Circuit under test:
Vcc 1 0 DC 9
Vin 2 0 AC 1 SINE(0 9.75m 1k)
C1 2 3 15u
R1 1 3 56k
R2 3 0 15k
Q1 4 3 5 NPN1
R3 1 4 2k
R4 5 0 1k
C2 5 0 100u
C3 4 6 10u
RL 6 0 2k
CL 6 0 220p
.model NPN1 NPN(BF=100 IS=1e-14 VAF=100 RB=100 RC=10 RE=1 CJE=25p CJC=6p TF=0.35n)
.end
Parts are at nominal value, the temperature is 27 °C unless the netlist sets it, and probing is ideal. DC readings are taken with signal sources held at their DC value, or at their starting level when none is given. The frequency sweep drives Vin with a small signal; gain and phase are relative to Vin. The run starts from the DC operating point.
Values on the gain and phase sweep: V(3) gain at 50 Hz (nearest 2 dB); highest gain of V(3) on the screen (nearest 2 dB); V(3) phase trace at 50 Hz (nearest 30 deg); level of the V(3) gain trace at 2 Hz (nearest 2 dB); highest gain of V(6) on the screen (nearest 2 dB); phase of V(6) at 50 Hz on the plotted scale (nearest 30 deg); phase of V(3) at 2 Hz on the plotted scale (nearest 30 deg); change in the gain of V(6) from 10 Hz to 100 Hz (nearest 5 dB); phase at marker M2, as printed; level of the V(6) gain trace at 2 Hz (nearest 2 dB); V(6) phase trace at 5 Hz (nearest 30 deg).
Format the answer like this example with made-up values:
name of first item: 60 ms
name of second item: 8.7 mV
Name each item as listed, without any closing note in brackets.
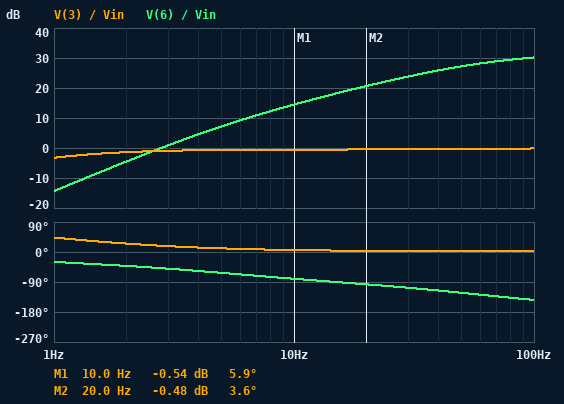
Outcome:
V(3) gain at 50 Hz: 0 dB
highest gain of V(3) on the screen: 0 dB
V(3) phase trace at 50 Hz: 0 deg
level of the V(3) gain trace at 2 Hz: -2 dB
highest gain of V(6) on the screen: 30 dB
phase of V(6) at 50 Hz on the plotted scale: -120 deg
phase of V(3) at 2 Hz on the plotted scale: 30 deg
change in the gain of V(6) from 10 Hz to 100 Hz: 15 dB
phase at marker M2, as printed: 3.6 deg
level of the V(6) gain trace at 2 Hz: -4 dB
V(6) phase trace at 5 Hz: -60 deg
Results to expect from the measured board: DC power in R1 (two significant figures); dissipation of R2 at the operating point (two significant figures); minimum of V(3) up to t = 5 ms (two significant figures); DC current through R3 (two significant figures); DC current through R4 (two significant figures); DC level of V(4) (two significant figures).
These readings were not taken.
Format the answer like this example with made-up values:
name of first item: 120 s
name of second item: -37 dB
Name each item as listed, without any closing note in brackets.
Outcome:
DC power in R1: 930 µW
dissipation of R2 at the operating point: 210 µW
minimum of V(3) up to t = 5 ms: 1.8 V
DC current through R3: 1.1 mA
DC current through R4: 1.1 mA
DC level of V(4): 6.8 V
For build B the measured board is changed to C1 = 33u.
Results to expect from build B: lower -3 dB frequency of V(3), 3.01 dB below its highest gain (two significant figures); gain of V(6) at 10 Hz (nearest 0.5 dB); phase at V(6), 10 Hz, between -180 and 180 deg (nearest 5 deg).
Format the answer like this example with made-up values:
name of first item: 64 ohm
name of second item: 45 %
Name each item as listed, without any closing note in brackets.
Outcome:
lower -3 dB frequency of V(3), 3.01 dB below its highest gain: 470 mHz
gain of V(6) at 10 Hz: 15.0 dB
phase at V(6), 10 Hz, between -180 and 180 deg: -85 deg
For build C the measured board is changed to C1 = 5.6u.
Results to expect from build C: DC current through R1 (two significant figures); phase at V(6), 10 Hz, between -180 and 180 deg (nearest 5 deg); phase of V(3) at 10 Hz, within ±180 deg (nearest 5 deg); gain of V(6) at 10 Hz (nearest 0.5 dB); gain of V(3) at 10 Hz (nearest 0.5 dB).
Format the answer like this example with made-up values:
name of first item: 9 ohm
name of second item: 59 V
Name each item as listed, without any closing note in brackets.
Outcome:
DC current through R1: 130 µA
phase at V(6), 10 Hz, between -180 and 180 deg: -70 deg
phase of V(3) at 10 Hz, within ±180 deg: 15 deg
gain of V(6) at 10 Hz: 13.5 dB
gain of V(3) at 10 Hz: -1.5 dB
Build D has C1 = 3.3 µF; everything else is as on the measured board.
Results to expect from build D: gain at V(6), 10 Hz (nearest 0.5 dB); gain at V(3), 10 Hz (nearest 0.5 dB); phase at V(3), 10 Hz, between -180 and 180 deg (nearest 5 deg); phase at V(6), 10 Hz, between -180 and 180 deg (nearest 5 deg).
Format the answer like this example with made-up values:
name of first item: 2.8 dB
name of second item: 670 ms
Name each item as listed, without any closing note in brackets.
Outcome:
gain at V(6), 10 Hz: 12.5 dB
gain at V(3), 10 Hz: -2.5 dB
phase at V(3), 10 Hz, between -180 and 180 deg: 20 deg
phase at V(6), 10 Hz, between -180 and 180 deg: -65 deg
